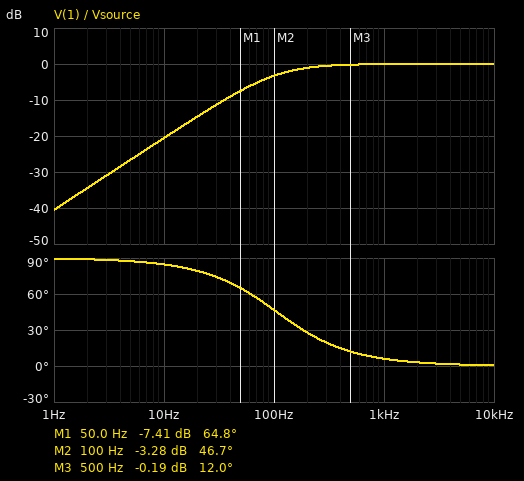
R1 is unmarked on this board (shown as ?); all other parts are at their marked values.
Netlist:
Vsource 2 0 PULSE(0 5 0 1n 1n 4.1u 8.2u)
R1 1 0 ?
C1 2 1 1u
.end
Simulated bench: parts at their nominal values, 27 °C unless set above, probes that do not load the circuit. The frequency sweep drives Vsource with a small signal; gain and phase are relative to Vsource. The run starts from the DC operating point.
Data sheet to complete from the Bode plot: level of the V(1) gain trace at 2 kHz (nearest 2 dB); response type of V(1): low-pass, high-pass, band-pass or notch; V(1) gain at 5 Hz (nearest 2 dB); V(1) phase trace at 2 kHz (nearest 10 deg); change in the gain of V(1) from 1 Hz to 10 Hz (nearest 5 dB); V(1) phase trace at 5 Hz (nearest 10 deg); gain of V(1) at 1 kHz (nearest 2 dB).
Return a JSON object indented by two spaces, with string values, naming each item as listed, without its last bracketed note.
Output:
{
  "level of the V(1) gain trace at 2 kHz": "0 dB",
  "response type of V(1): low-pass, high-pass, band-pass or notch": "high-pass",
  "V(1) gain at 5 Hz": "-26 dB",
  "V(1) phase trace at 2 kHz": "0 deg",
  "change in the gain of V(1) from 1 Hz to 10 Hz": "20 dB",
  "V(1) phase trace at 5 Hz": "90 deg",
  "gain of V(1) at 1 kHz": "0 dB"
}
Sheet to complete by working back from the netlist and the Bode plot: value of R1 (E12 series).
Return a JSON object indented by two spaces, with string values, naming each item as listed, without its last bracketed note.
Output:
{
  "value of R1": "1.5 kΩ"
}
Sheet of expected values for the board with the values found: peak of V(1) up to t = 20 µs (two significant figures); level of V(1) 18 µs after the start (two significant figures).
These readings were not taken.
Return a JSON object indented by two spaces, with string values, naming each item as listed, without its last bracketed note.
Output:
{
  "peak of V(1) up to t = 20 µs": "5.0 V",
  "level of V(1) 18 µs after the start": "5.0 V"
}
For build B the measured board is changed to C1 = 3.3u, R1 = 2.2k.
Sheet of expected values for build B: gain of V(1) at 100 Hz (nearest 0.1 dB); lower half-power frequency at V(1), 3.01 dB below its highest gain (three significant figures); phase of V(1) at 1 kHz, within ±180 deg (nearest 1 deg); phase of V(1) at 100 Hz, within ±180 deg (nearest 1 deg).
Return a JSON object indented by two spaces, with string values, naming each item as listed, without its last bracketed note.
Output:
{
  "gain of V(1) at 100 Hz": "-0.2 dB",
  "lower half-power frequency at V(1), 3.01 dB below its highest gain": "21.9 Hz",
  "phase of V(1) at 1 kHz, within ±180 deg": "1 deg",
  "phase of V(1) at 100 Hz, within ±180 deg": "12 deg"
}
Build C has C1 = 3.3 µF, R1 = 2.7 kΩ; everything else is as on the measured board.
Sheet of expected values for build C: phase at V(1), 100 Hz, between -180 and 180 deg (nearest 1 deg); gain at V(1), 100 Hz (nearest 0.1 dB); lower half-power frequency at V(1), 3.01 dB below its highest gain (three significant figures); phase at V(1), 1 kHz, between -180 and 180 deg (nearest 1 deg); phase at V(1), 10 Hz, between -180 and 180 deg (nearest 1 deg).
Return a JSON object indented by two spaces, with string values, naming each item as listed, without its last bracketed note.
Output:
{
  "phase at V(1), 100 Hz, between -180 and 180 deg": "10 deg",
  "gain at V(1), 100 Hz": "-0.1 dB",
  "lower half-power frequency at V(1), 3.01 dB below its highest gain": "17.9 Hz",
  "phase at V(1), 1 kHz, between -180 and 180 deg": "1 deg",
  "phase at V(1), 10 Hz, between -180 and 180 deg": "61 deg"
}
